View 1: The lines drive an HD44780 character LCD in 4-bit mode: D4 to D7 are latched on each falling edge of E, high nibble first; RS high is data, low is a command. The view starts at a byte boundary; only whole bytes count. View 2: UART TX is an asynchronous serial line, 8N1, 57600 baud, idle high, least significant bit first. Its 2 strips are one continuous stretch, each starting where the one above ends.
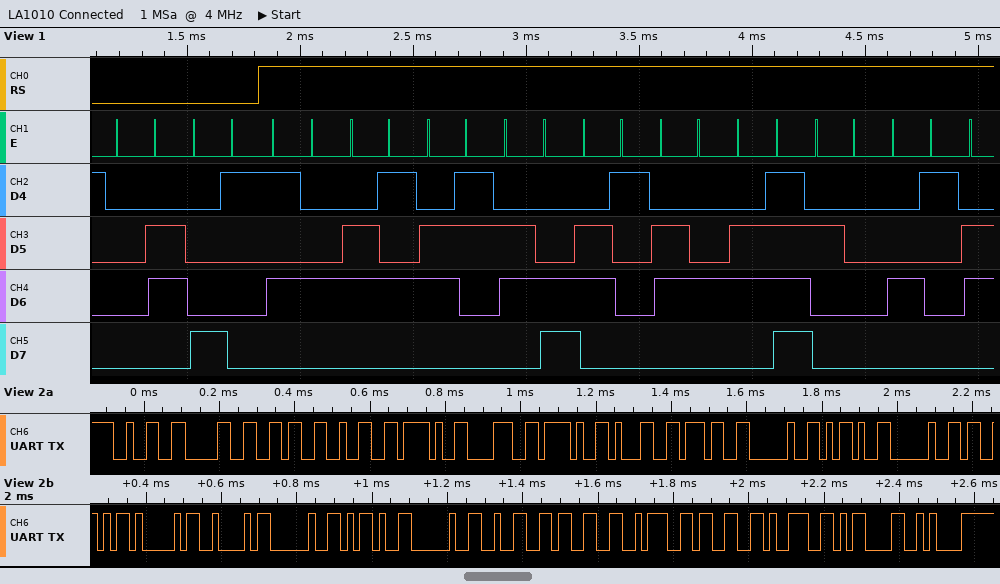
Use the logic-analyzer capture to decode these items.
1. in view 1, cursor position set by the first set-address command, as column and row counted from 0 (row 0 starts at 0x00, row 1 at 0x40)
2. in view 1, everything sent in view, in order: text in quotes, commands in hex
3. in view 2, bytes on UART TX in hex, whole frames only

column 1, row 0
0x06 0x81 "Teclado A"
0x32 0x30 0x36 0x32 0x2F 0x38 0x2F 0x31 0x37 0x20 0x2D 0x20 0x53 0x41 0x42 0x20 0x2D 0x20 0x32 0x33 0x3A 0x33 0x39 0x0D 0x0A
